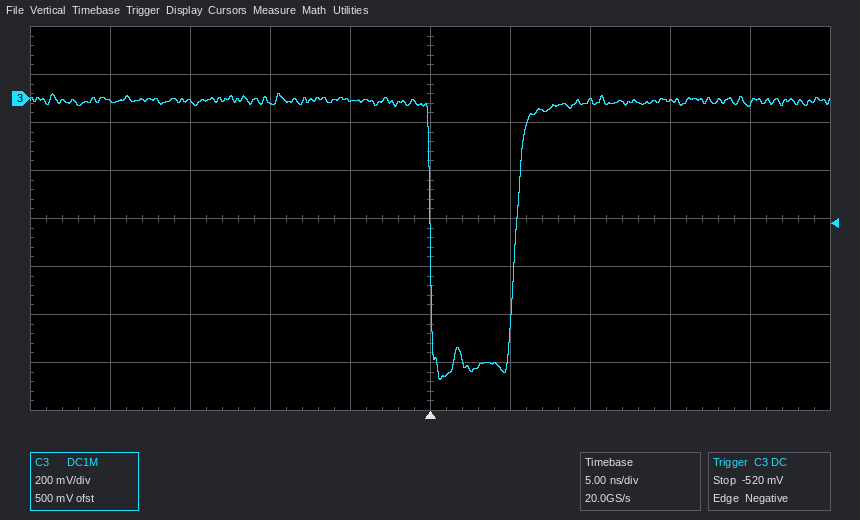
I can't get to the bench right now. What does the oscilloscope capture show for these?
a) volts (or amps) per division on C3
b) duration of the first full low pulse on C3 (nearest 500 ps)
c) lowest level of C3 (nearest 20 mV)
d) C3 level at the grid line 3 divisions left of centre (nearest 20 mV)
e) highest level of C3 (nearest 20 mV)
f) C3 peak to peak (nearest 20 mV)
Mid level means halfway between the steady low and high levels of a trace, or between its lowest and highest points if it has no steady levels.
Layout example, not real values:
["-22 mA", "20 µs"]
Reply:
["200 mV", "5.5 ns", "-1.18 V", "-20 mV", "20 mV", "1.20 V"]
